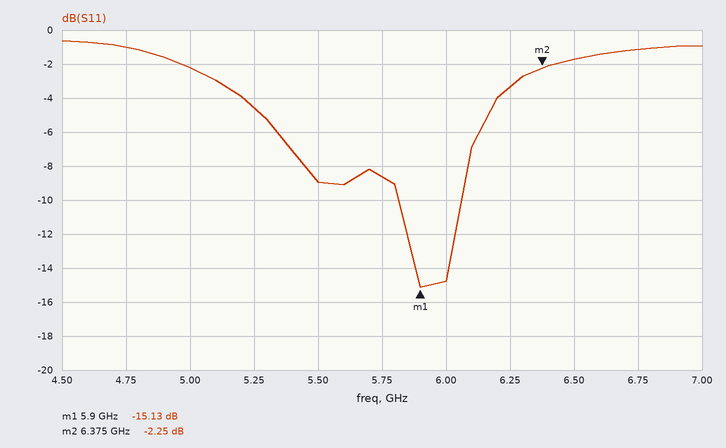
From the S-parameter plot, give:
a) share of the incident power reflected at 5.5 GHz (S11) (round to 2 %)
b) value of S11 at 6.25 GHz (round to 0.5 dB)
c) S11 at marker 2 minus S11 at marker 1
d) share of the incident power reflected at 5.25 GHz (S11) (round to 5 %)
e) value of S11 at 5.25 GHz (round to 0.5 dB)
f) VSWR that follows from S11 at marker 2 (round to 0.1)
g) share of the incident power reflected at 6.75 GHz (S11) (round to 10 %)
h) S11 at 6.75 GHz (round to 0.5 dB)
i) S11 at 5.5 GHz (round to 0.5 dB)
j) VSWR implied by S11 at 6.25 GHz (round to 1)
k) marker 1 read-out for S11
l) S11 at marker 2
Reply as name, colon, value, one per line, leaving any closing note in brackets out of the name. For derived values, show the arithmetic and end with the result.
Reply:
share of the incident power reflected at 5.5 GHz (S11): 10^(-9/10) ≈ 12.6 %, so 12 % to the nearest 2 %
value of S11 at 6.25 GHz: -3.5 dB
S11 at marker 2 minus S11 at marker 1: -2.25 − (-15.13) = 12.88 dB
share of the incident power reflected at 5.25 GHz (S11): 10^(-4.5/10) ≈ 35 %
value of S11 at 5.25 GHz: -4.5 dB
VSWR that follows from S11 at marker 2: (1 + 0.7718)/(1 − 0.7718) ≈ 7.8
share of the incident power reflected at 6.75 GHz (S11): 10^(-1/10) ≈ 79.4 %, so 80 % to the nearest 10 %
S11 at 6.75 GHz: -1.0 dB
S11 at 5.5 GHz: -9.0 dB
VSWR implied by S11 at 6.25 GHz: |Γ| = 10^(-3.5/20) = 0.6683; VSWR = (1 + 0.6683)/(1 − 0.6683) ≈ 5
marker 1 read-out for S11: -15.13 dB
S11 at marker 2: -2.25 dB
